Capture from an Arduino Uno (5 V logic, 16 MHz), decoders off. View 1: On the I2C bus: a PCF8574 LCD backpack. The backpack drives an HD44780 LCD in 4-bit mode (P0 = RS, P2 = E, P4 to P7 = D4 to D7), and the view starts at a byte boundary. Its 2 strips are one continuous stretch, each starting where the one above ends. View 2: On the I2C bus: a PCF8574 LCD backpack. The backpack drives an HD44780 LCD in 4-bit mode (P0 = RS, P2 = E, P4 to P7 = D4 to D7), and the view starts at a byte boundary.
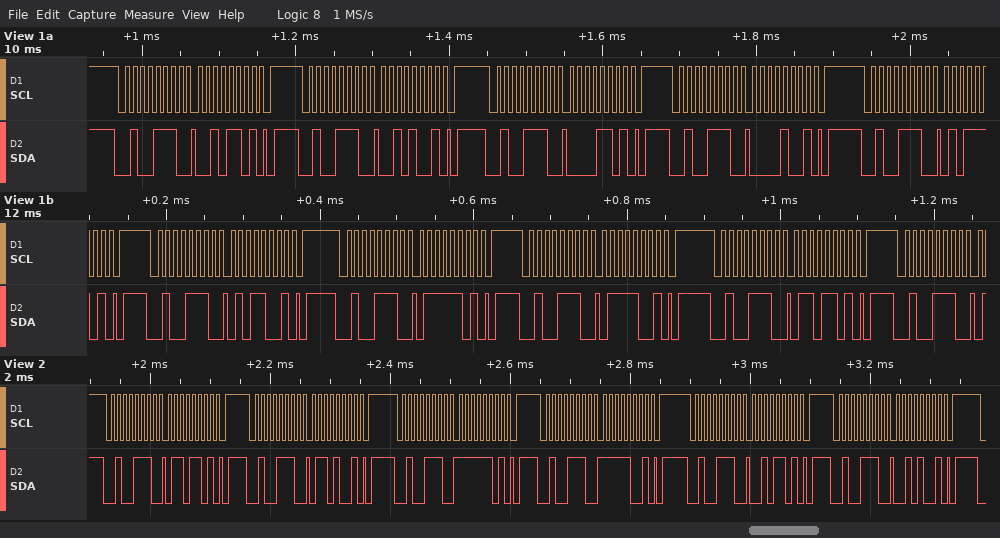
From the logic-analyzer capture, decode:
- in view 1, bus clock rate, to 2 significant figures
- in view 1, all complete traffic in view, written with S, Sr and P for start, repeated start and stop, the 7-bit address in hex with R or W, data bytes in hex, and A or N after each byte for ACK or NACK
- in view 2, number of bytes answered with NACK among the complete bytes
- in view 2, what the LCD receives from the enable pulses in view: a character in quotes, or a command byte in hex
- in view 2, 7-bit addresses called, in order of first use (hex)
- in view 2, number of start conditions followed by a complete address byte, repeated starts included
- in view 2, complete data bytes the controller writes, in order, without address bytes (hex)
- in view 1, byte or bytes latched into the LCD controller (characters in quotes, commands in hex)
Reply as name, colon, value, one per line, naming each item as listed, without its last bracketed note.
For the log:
in view 1, bus clock rate, to 2 significant figures: 100 kHz
in view 1, all complete traffic in view, written with S, Sr and P for start, repeated start and stop, the 7-bit address in hex with R or W, data bytes in hex, and A or N after each byte for ACK or NACK: S 27W A 2D A P S 27W A 29 A P S 27W A 0D A P S 27W A 09 A P S 27W A 5D A P S 27W A 59 A P S 27W A 7D A P S 27W A 79 A P S 27W A 6D A P S 27W A
in view 2, number of bytes answered with NACK among the complete bytes: 0
in view 2, what the LCD receives from the enable pulses in view: a character in quotes, or a command byte in hex: 'o'
in view 2, 7-bit addresses called, in order of first use: 0x27
in view 2, number of start conditions followed by a complete address byte, repeated starts included: 6
in view 2, complete data bytes the controller writes, in order, without address bytes: 6D 69 FD F9 2D 29
in view 1, byte or bytes latched into the LCD controller: ' ' 'W'
